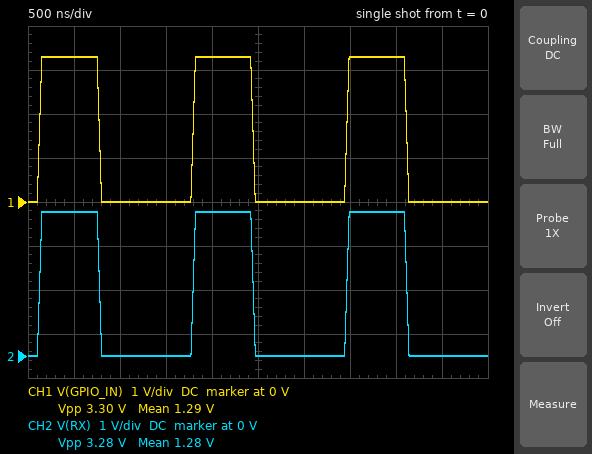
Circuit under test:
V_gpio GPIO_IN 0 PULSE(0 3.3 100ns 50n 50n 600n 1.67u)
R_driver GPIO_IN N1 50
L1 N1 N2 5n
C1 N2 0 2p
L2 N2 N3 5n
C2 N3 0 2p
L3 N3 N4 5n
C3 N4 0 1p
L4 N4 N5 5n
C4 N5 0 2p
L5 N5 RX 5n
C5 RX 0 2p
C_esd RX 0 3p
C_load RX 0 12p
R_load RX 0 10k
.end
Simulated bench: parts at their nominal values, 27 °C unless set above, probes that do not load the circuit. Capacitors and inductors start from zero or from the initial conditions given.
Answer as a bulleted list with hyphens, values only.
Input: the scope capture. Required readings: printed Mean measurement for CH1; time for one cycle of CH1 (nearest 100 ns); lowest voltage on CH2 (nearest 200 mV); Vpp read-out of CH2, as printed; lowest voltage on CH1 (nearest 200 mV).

- 1.29 V
- 1.7 µs
- 0 V
- 3.28 V
- 0 V
